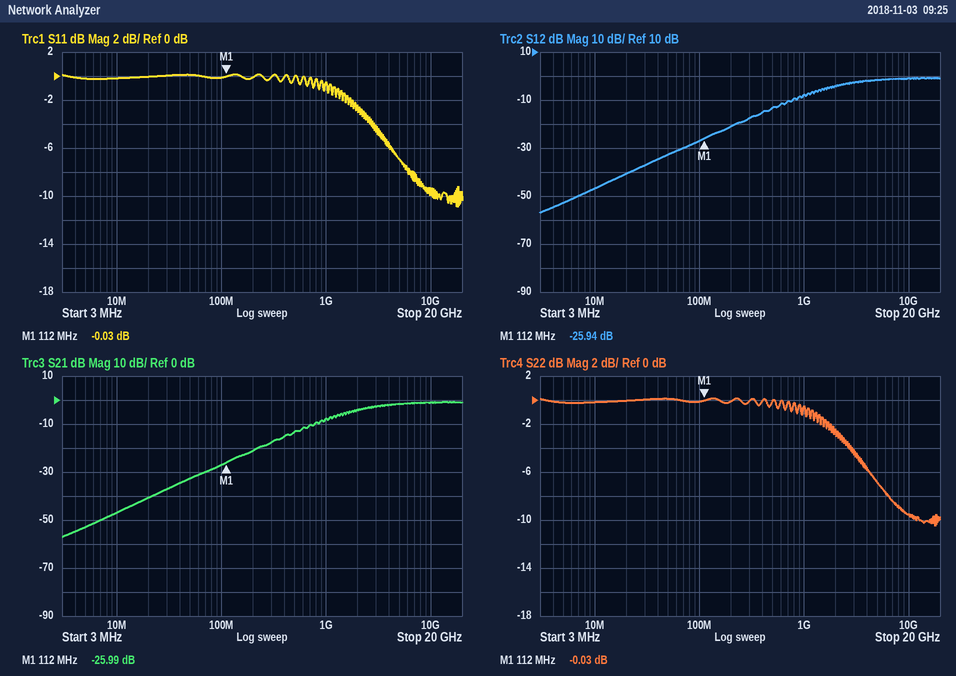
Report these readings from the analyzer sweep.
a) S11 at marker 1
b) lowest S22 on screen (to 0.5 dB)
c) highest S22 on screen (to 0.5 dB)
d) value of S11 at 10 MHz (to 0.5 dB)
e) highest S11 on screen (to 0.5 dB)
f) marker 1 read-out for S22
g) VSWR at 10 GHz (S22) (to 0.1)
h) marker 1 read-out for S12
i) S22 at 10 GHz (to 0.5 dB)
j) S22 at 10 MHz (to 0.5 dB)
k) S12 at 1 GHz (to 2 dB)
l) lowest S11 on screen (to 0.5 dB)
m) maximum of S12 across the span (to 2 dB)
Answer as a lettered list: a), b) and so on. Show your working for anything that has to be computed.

a) -0.03 dB
b) -10.5 dB
c) 0.0 dB
d) 0.0 dB
e) 0.0 dB
f) -0.03 dB
g) |Γ| = 10^(-9.5/20) = 0.3350; VSWR = (1 + 0.3350)/(1 − 0.3350) ≈ 2.0
h) -25.94 dB
i) -9.5 dB
j) 0.0 dB
k) -8 dB
l) -11.0 dB
m) 0 dB
